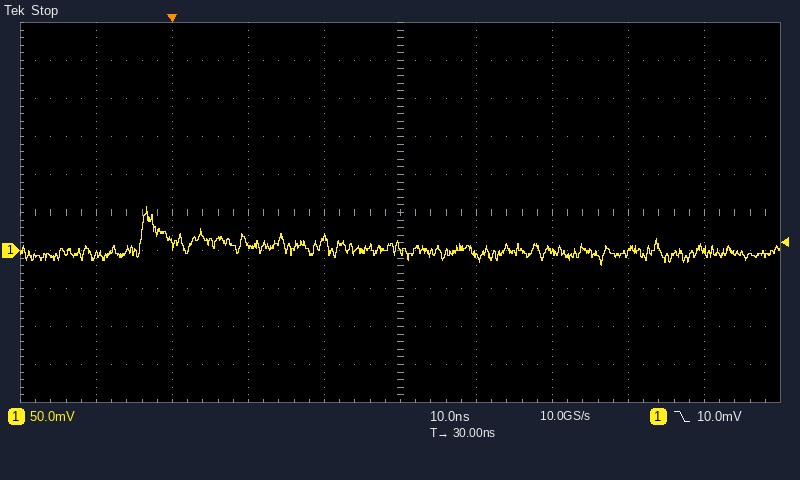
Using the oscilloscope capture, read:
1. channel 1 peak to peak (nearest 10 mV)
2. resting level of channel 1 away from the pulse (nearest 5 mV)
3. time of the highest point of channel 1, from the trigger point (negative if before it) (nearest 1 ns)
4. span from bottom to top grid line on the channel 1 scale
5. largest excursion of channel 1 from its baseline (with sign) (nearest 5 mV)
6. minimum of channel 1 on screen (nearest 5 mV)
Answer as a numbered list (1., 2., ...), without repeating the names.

1. 80 mV
2. 0 mV
3. -3 ns
4. 500 mV
5. +60 mV
6. -20 mV
